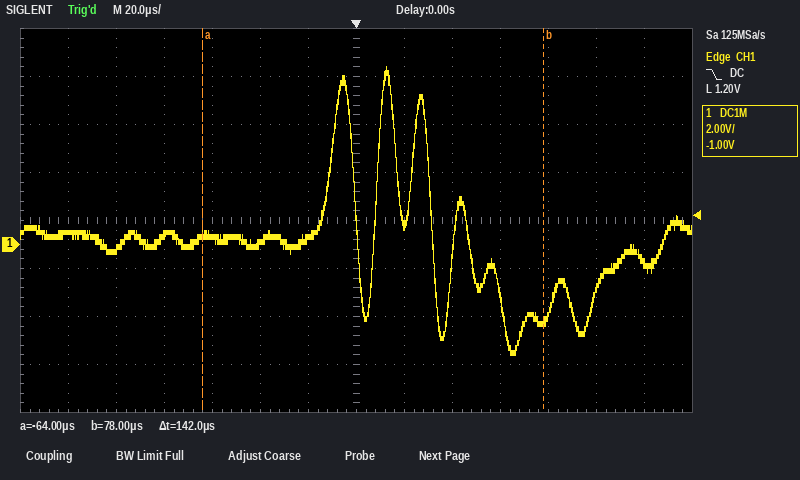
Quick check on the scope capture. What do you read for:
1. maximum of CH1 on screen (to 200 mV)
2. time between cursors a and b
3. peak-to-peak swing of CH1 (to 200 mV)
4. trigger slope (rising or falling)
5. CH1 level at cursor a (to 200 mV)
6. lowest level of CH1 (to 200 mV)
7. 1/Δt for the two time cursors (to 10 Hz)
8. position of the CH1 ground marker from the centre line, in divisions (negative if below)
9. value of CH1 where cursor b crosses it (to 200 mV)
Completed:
7.4 V
142 µs
12.0 V
falling
400 mV
-4.6 V
7.04 kHz
-0.5 div
-3.2 V
